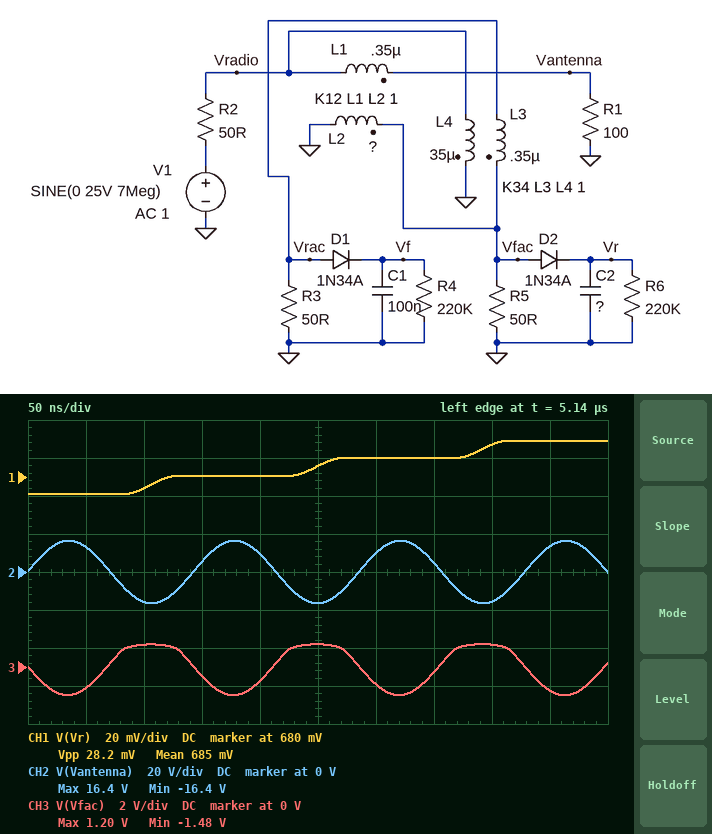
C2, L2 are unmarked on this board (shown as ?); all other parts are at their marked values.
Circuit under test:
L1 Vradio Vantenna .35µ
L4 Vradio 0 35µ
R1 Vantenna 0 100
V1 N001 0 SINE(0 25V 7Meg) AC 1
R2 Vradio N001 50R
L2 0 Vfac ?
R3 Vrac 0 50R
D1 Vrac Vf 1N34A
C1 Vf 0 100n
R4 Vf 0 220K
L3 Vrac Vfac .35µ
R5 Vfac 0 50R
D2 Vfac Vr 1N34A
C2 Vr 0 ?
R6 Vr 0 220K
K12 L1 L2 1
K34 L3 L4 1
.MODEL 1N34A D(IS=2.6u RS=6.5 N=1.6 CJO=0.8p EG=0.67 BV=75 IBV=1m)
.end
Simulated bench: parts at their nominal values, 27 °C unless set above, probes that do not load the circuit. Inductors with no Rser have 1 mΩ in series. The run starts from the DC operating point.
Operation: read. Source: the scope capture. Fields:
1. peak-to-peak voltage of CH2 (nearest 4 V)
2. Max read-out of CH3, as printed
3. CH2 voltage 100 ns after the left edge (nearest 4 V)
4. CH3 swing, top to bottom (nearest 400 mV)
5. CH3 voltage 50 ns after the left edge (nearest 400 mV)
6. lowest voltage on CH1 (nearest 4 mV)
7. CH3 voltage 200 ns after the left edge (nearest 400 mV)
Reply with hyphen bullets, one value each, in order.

- 32 V
- 1.20 V
- -16 V
- 2.8 V
- -1.2 V
- 672 mV
- -800 mV
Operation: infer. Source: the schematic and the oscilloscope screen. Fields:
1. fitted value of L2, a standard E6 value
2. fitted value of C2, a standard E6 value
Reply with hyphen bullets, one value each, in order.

- 10 µH
- 68 nF
